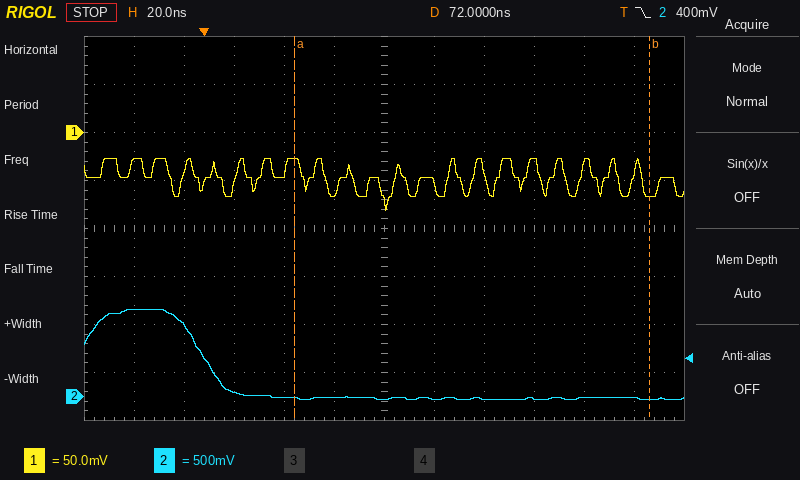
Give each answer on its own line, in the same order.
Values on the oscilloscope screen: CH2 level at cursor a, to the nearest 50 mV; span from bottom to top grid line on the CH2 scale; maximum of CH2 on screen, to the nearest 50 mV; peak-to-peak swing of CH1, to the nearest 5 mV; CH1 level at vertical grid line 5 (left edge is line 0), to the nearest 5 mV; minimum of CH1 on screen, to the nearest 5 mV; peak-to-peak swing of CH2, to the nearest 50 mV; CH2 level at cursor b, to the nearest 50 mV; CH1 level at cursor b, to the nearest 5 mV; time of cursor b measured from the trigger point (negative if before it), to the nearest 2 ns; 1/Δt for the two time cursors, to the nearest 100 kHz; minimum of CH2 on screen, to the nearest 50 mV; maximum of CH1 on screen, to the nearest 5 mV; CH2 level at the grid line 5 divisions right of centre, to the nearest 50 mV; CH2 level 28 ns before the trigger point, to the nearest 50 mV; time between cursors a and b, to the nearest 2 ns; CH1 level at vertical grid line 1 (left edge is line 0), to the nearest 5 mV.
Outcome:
0 mV
4 V
900 mV
55 mV
-65 mV
-80 mV
950 mV
-50 mV
-65 mV
+178 ns
7.0 MHz
-50 mV
-25 mV
0 mV
900 mV
142 ns
-30 mV
